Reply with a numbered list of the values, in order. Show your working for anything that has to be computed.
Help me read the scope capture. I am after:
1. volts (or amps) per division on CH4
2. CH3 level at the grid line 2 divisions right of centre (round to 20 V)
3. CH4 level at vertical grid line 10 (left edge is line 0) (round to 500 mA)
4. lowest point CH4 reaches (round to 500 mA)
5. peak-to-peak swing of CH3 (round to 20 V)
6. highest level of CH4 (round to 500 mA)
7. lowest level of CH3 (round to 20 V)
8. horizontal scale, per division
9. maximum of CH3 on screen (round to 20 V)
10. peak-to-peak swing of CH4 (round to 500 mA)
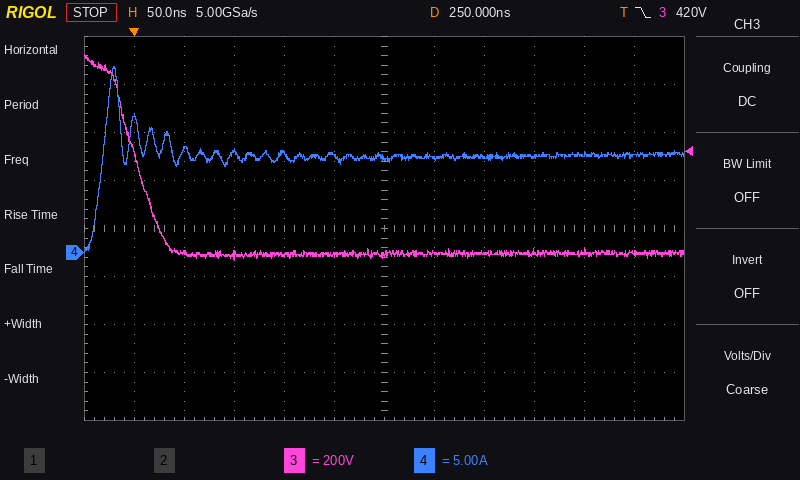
1. 5 A
2. 0 V
3. 10.0 A
4. 0.0 A
5. 820 V − (-40 V) = 860 V
6. 19.5 A
7. -40 V
8. 50 ns
9. 820 V
10. 19.5 A − (0.0 A) = 19.5 A
